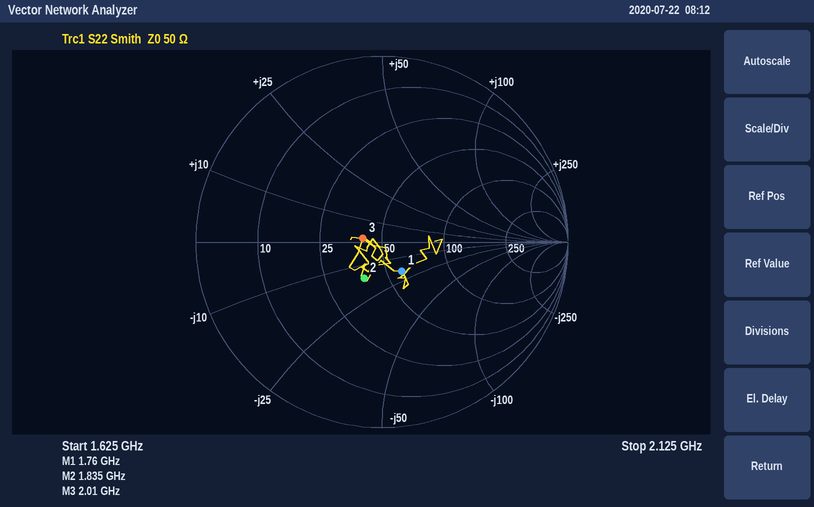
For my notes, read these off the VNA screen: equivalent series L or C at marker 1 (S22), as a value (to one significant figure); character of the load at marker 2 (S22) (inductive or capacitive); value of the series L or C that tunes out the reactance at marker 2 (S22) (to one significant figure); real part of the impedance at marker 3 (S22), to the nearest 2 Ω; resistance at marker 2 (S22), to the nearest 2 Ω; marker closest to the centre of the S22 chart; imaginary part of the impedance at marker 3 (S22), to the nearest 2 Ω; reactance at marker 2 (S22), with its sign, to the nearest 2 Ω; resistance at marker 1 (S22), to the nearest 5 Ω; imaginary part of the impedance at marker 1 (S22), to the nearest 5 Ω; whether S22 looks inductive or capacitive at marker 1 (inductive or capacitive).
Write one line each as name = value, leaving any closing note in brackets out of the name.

equivalent series L or C at marker 1 (S22), as a value = 5 pF
character of the load at marker 2 (S22) = capacitive
value of the series L or C that tunes out the reactance at marker 2 (S22) = 1 nH
real part of the impedance at marker 3 (S22), to the nearest 2 Ω = 40 Ω
resistance at marker 2 (S22), to the nearest 2 Ω = 38 Ω
marker closest to the centre of the S22 chart = marker 3
imaginary part of the impedance at marker 3 (S22), to the nearest 2 Ω = +2 Ω
reactance at marker 2 (S22), with its sign, to the nearest 2 Ω = -16 Ω
resistance at marker 1 (S22), to the nearest 5 Ω = 60 Ω
imaginary part of the impedance at marker 1 (S22), to the nearest 5 Ω = -20 Ω
whether S22 looks inductive or capacitive at marker 1 = capacitive
